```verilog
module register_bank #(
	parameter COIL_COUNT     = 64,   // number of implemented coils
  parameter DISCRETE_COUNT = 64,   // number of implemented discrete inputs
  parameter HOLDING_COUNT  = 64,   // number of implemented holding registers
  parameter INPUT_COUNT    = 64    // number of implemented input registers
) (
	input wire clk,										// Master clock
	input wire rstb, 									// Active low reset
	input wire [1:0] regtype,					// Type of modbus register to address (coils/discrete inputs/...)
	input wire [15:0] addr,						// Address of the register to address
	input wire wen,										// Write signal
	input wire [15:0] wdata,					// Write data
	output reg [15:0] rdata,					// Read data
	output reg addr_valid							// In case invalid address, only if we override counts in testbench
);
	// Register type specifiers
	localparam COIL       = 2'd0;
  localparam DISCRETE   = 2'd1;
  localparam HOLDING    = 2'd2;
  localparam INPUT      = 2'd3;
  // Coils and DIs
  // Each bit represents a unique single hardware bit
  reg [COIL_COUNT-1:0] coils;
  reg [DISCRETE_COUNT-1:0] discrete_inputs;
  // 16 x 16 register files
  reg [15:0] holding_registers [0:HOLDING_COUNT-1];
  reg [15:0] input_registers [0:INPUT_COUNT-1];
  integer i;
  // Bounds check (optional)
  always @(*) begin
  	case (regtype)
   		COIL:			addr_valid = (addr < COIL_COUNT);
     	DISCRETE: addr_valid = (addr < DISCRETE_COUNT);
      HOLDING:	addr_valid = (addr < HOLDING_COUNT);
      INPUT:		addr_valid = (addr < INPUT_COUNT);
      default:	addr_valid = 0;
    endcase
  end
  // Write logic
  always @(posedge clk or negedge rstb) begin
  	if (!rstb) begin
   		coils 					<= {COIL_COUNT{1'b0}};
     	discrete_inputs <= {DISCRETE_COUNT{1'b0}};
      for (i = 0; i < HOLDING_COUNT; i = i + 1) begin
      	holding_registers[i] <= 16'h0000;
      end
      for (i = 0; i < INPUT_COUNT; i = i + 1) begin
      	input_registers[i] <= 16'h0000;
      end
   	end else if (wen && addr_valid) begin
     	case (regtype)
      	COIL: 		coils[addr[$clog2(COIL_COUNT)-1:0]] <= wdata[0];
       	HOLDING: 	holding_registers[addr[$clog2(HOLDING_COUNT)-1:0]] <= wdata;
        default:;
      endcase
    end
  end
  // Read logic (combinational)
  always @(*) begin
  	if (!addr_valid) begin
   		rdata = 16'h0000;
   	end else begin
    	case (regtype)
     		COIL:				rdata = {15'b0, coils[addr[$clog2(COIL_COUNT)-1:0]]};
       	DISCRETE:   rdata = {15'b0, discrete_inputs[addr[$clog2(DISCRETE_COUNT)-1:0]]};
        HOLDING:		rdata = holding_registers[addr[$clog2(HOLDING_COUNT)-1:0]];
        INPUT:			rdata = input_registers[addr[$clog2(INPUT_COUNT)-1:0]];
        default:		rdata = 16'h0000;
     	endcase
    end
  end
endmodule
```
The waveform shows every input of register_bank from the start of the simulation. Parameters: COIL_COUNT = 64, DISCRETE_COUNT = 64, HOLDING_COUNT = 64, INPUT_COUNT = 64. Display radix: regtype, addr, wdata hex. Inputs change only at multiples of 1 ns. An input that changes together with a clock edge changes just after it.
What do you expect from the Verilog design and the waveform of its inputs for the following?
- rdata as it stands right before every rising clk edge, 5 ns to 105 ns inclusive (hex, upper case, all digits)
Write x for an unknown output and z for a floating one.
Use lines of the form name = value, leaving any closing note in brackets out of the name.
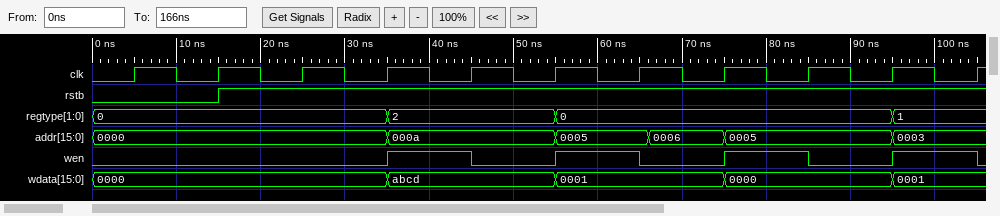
rdata as it stands right before every rising clk edge, 5 ns to 105 ns inclusive = 0000, 0000, 0000, 0000, 0000, ABCD, 0000, 0000, 0001, 0000, 0000
